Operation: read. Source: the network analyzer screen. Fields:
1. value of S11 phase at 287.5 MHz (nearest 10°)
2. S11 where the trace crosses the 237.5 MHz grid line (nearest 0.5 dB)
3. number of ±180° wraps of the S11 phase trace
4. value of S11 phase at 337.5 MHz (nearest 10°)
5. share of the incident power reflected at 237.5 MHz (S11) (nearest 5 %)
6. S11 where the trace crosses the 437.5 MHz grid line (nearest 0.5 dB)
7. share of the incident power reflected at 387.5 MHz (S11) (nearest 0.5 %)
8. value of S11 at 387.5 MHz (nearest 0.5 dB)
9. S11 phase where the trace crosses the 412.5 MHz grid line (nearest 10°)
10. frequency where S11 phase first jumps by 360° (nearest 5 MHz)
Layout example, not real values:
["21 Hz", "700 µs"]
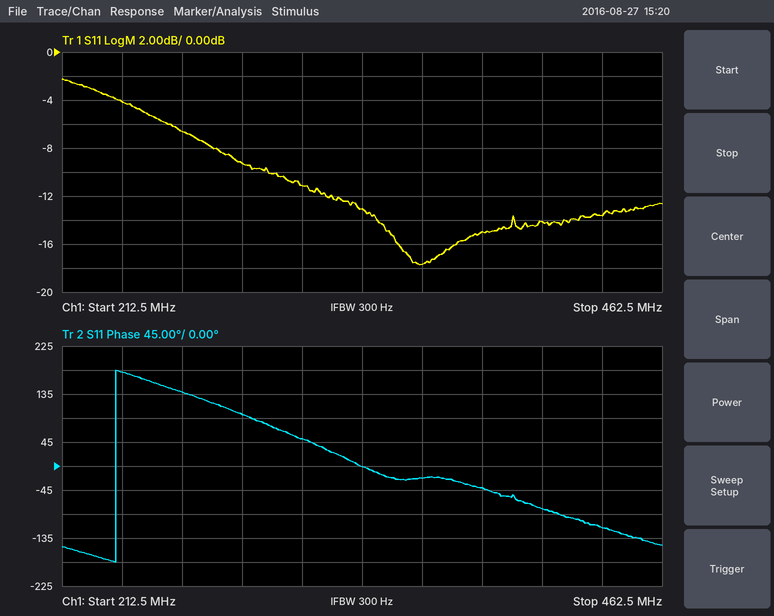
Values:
["100°", "-4.0 dB", "1", "0°", "40 %", "-13.5 dB", "3.0 %", "-15.0 dB", "-80°", "235 MHz"]
